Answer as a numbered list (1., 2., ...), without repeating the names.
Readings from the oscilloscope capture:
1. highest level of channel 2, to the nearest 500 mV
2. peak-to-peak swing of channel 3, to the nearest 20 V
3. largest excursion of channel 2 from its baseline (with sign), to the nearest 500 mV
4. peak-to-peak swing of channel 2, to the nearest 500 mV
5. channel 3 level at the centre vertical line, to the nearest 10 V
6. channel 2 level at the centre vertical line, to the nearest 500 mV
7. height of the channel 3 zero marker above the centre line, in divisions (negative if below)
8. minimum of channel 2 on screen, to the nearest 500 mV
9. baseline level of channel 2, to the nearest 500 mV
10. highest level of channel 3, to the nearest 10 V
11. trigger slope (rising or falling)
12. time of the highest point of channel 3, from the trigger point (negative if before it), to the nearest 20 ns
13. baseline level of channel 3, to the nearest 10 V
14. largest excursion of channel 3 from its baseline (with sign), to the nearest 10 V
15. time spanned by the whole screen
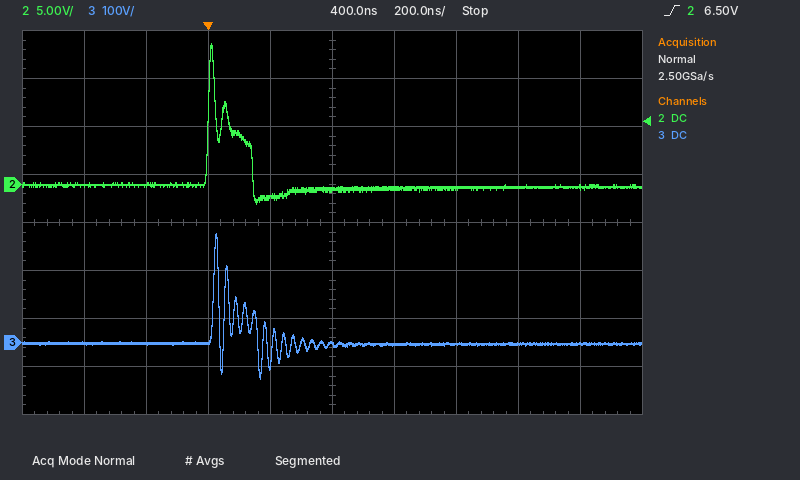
1. 14.5 V
2. 300 V
3. +15.0 V
4. 16.5 V
5. 0 V
6. -500 mV
7. -2.5 div
8. -2.0 V
9. -500 mV
10. 230 V
11. rising
12. +20 ns
13. 0 V
14. +230 V
15. 2 µs
